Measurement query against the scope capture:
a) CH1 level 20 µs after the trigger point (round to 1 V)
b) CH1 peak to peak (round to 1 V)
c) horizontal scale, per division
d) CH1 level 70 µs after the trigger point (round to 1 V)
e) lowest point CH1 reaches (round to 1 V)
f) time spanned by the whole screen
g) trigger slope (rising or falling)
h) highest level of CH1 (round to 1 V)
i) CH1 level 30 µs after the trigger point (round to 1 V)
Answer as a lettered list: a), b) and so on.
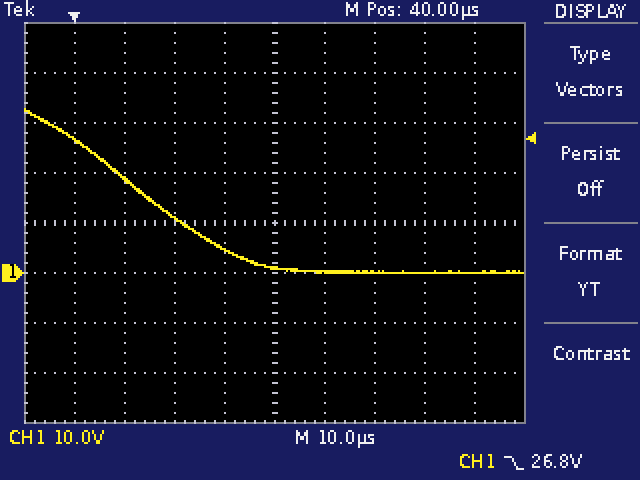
a) 11 V
b) 33 V
c) 10 µs
d) 0 V
e) 0 V
f) 100 µs
g) falling
h) 33 V
i) 5 V
